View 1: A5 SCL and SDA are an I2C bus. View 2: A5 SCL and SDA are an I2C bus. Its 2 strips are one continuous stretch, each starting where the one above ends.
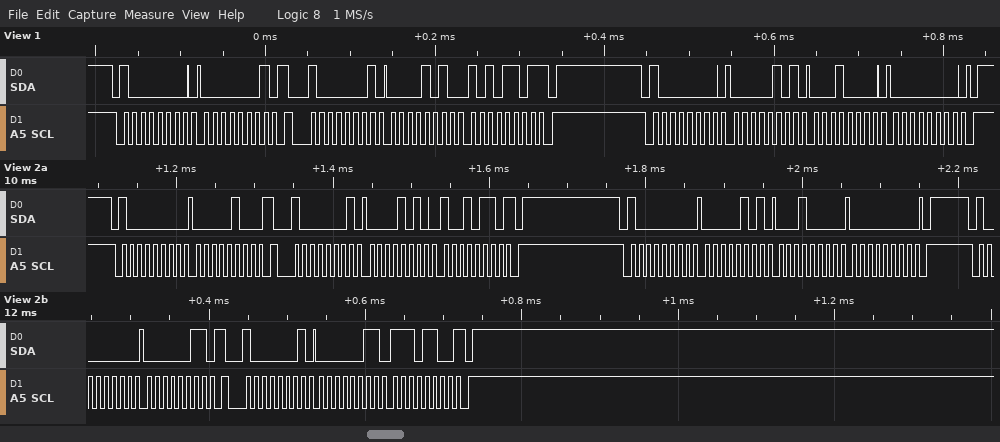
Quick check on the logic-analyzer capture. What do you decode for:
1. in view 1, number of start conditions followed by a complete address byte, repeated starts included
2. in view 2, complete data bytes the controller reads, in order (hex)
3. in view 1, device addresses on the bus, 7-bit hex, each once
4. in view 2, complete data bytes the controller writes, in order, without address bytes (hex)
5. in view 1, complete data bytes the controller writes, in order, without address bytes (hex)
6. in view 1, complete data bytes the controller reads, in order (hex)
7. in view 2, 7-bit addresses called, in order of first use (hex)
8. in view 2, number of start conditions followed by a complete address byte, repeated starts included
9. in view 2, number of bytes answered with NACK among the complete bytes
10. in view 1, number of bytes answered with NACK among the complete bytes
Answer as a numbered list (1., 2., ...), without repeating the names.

1. 3
2. 0A 96 03 EC
3. 0x40
4. 04 05 10 00 03
5. 01 05 10 00
6. 0A AD
7. 0x40
8. 5
9. 2
10. 1
